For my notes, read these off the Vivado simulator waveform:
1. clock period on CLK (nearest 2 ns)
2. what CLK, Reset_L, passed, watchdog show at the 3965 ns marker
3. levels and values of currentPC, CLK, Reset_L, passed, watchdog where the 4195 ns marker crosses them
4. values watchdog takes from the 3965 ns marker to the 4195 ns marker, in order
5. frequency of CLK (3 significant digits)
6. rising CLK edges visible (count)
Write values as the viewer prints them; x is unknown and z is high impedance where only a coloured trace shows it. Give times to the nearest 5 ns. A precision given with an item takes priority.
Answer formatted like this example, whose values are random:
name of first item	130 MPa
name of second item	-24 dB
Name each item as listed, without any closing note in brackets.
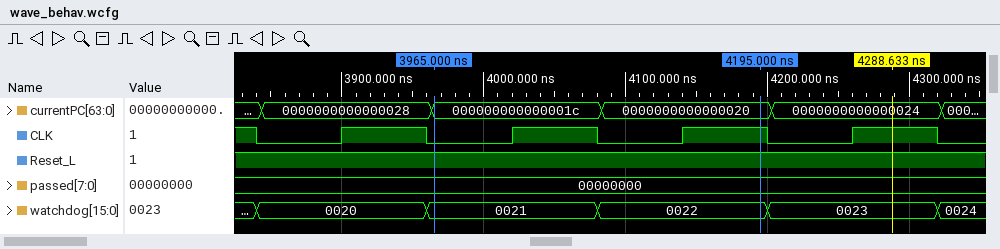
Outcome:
clock period on CLK	120 ns
what CLK, Reset_L, passed, watchdog show at the 3965 ns marker	CLK=0, Reset_L=1, passed=00000000, watchdog=0021
levels and values of currentPC, CLK, Reset_L, passed, watchdog where the 4195 ns marker crosses them	currentPC=0000000000000020, CLK=1, Reset_L=1, passed=00000000, watchdog=0022
values watchdog takes from the 3965 ns marker to the 4195 ns marker, in order	0021, 0022
frequency of CLK	8.33 MHz
rising CLK edges visible	4
